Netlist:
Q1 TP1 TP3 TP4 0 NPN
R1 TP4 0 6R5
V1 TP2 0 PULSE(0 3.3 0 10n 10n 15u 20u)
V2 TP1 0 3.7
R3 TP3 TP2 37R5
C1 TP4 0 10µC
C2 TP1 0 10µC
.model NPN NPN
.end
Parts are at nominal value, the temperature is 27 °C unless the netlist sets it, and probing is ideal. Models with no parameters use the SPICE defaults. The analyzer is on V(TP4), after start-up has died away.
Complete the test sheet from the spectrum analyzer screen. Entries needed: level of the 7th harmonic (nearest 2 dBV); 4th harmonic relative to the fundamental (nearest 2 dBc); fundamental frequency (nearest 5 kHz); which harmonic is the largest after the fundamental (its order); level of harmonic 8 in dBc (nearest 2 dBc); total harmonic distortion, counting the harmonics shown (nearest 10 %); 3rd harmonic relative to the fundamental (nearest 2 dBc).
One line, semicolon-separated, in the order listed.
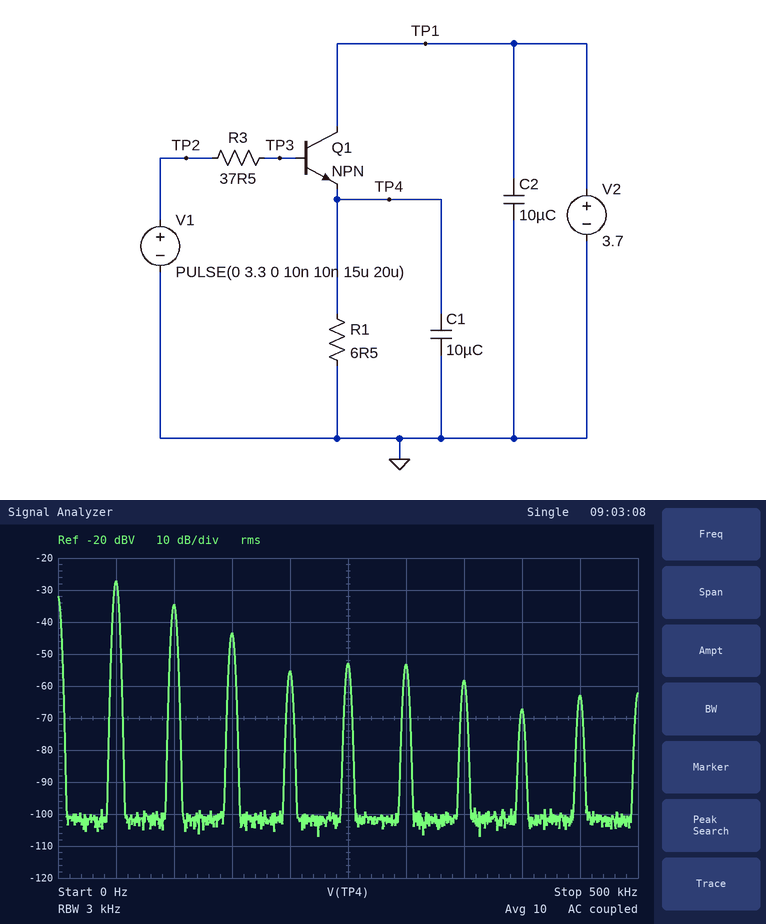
-58 dBV; -28 dBc; 50 kHz; 2; -40 dBc; 50 %; -16 dBc
